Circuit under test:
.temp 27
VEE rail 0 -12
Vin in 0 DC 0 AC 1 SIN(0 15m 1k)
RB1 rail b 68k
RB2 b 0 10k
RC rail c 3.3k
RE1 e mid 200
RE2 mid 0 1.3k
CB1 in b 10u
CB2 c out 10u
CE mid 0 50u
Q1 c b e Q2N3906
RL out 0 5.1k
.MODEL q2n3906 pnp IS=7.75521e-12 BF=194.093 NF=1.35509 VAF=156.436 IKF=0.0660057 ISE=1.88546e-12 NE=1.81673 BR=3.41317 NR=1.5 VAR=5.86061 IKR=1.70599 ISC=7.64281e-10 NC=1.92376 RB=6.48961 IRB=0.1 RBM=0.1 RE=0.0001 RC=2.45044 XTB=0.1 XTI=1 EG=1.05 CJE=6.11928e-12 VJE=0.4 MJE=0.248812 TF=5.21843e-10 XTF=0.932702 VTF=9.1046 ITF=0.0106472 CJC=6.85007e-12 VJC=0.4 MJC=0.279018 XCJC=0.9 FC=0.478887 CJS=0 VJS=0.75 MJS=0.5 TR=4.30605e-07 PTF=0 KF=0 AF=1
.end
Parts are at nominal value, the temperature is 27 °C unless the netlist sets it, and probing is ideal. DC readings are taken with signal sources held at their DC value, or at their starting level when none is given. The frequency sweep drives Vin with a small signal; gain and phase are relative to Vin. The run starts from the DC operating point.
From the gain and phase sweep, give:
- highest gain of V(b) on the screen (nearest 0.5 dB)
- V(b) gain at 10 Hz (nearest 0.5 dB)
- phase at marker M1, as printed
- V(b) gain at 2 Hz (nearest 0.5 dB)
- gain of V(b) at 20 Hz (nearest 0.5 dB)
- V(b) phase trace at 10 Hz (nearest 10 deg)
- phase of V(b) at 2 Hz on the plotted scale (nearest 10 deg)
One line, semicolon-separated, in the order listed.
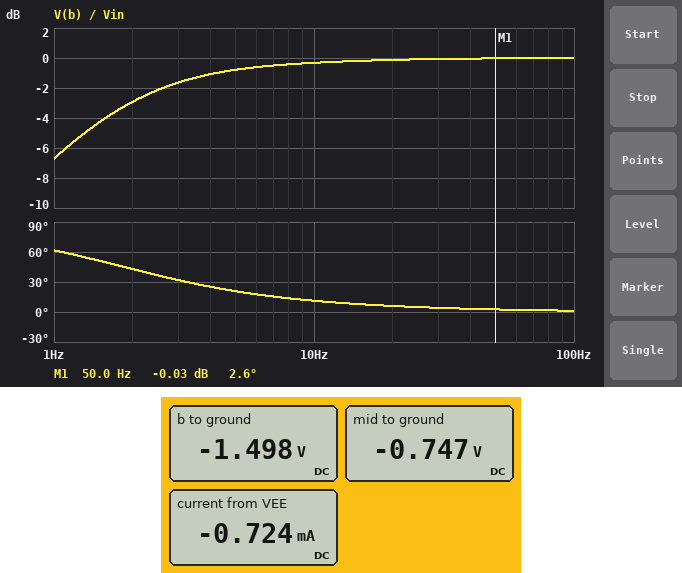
0 dB; -0.5 dB; 2.6 deg; -3.0 dB; 0 dB; 10 deg; 40 deg
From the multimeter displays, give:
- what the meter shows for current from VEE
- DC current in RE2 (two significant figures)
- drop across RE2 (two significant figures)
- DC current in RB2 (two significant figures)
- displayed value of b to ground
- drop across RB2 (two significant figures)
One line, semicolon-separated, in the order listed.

-0.724 mA; 570 µA; 750 mV; 150 µA; -1.498 V; 1.5 V
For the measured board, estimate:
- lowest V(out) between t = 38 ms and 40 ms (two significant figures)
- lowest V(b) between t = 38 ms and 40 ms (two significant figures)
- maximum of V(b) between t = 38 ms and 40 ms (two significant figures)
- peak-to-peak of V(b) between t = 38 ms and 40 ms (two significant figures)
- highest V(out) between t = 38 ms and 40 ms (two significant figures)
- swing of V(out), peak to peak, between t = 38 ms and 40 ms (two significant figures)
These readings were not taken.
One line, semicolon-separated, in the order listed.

-110 mV; -1.5 V; -1.5 V; 30 mV; 110 mV; 230 mV
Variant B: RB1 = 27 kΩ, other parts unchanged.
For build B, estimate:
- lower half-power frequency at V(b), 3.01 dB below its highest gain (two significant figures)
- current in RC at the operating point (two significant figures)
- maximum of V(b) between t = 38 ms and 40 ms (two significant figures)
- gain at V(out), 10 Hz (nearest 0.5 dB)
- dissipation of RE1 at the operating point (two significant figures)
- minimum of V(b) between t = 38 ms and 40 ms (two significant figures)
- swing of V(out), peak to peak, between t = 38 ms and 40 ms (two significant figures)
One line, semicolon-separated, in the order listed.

2.3 Hz; 1.6 mA; -3.1 V; 13.0 dB; 540 µW; -3.2 V; 270 mV
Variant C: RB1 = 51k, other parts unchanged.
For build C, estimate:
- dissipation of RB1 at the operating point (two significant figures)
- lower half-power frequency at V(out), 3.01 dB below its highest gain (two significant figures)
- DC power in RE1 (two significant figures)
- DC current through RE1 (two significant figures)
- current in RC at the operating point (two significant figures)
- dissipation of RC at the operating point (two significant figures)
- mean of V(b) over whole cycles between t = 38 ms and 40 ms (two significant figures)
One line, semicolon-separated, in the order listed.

2.0 mW; 16 Hz; 140 µW; 840 µA; 830 µA; 2.3 mW; -1.9 V
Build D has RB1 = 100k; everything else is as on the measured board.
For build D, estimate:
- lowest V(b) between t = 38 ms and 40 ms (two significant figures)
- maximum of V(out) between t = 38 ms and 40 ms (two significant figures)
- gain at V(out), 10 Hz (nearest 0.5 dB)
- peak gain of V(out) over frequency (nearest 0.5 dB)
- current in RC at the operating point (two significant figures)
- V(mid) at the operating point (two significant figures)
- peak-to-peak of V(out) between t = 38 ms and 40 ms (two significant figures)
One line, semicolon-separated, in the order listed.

-1.1 V; 95 mV; 11.5 dB; 16.0 dB; 300 µA; -390 mV; 190 mV
